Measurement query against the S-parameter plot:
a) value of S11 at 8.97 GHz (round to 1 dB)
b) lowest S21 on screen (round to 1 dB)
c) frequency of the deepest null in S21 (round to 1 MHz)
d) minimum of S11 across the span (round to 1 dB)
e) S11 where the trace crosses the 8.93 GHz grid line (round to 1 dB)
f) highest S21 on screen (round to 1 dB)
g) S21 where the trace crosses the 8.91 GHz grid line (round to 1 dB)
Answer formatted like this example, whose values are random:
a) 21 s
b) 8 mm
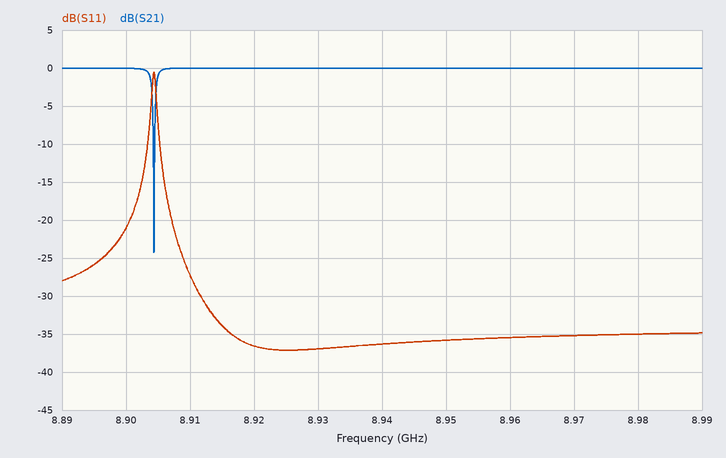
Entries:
a) -35 dB
b) -24 dB
c) 8.904 GHz
d) -37 dB
e) -37 dB
f) 0 dB
g) 0 dB
